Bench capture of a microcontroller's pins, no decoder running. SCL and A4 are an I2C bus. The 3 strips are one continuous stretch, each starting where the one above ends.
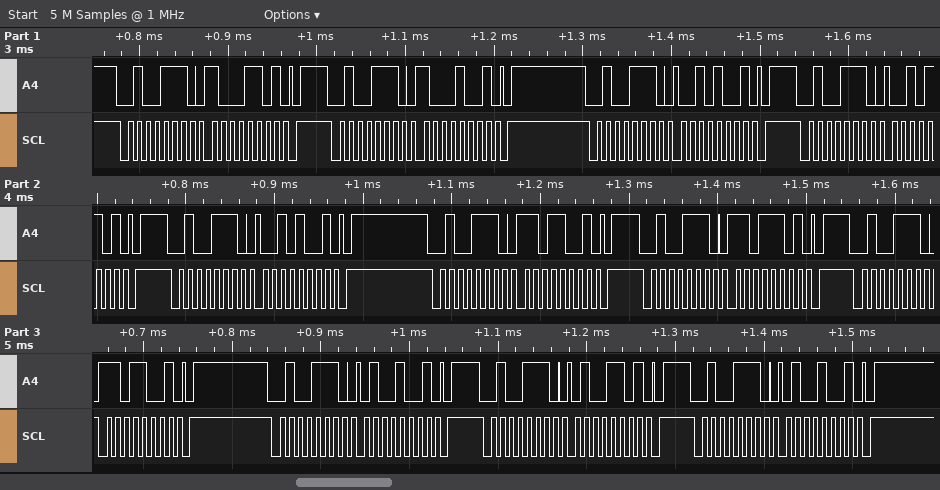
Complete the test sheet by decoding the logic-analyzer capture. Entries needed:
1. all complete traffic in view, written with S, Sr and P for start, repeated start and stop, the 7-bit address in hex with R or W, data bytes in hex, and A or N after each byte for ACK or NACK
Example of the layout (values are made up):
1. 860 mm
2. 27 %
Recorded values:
1. S 27W A 8D A P S 27W A 89 A P S 27W A 29 A P S 27W A 2D A P S 27W A 29 A P S 27W A D9 A P S 27W A DD A P S 27W A D9 A P S 27W A 49 A P S 27W A 4D A P S 27W A 49 A P
